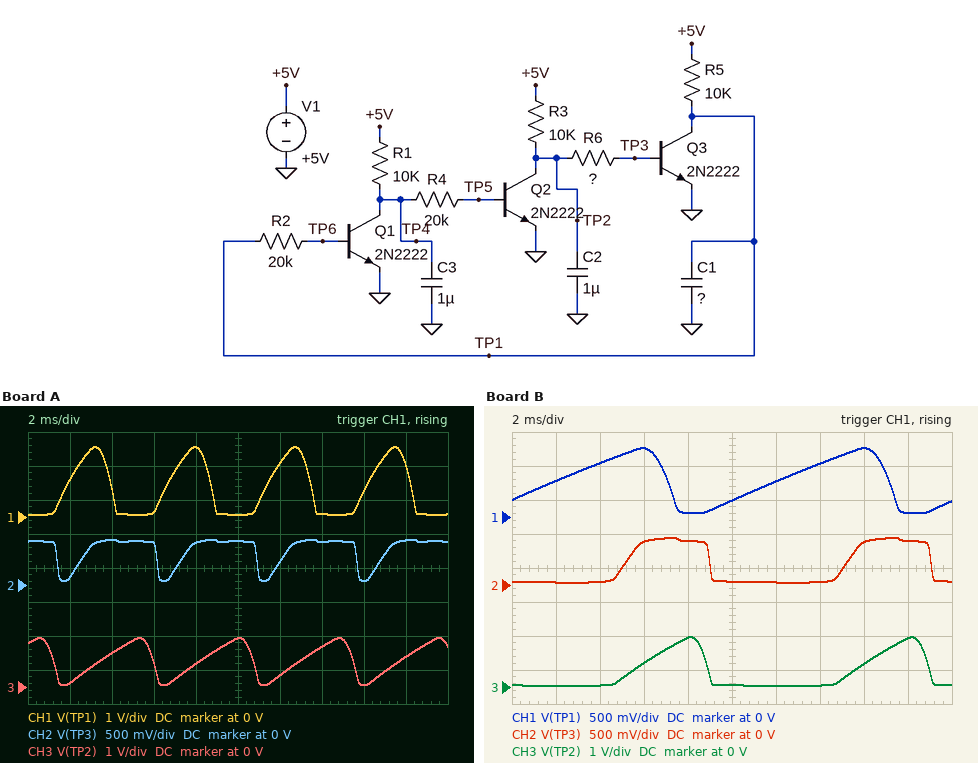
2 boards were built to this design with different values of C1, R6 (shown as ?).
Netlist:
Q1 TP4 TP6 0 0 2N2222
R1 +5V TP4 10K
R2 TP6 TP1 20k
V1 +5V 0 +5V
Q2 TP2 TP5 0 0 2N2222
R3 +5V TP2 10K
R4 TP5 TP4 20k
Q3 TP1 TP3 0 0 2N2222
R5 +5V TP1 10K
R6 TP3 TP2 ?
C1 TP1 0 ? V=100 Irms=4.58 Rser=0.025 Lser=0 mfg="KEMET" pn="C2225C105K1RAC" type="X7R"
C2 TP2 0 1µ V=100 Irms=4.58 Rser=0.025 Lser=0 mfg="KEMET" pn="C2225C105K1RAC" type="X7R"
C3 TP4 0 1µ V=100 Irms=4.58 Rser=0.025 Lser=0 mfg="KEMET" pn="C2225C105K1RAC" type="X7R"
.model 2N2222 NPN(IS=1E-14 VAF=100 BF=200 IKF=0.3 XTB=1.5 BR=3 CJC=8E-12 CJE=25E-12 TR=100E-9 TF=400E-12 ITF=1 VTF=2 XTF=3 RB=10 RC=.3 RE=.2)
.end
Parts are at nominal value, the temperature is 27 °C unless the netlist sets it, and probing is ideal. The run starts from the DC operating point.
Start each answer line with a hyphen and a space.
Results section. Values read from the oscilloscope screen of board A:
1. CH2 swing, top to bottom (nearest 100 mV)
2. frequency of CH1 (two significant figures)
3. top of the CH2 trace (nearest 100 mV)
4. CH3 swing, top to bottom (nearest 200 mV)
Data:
- 600 mV
- 210 Hz
- 700 mV
- 1.4 V
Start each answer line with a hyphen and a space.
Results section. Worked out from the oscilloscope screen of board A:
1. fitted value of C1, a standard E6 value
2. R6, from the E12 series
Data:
- 330 nF
- 47 kΩ
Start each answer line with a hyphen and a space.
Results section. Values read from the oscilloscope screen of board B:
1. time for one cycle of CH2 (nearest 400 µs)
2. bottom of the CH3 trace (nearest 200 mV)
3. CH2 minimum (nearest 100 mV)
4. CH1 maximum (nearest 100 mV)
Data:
- 10.0 ms
- 0 V
- 0 V
- 1.0 V
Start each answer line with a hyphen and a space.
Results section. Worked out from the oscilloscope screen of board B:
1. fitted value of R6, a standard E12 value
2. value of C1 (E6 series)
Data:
- 27 kΩ
- 3.3 µF
